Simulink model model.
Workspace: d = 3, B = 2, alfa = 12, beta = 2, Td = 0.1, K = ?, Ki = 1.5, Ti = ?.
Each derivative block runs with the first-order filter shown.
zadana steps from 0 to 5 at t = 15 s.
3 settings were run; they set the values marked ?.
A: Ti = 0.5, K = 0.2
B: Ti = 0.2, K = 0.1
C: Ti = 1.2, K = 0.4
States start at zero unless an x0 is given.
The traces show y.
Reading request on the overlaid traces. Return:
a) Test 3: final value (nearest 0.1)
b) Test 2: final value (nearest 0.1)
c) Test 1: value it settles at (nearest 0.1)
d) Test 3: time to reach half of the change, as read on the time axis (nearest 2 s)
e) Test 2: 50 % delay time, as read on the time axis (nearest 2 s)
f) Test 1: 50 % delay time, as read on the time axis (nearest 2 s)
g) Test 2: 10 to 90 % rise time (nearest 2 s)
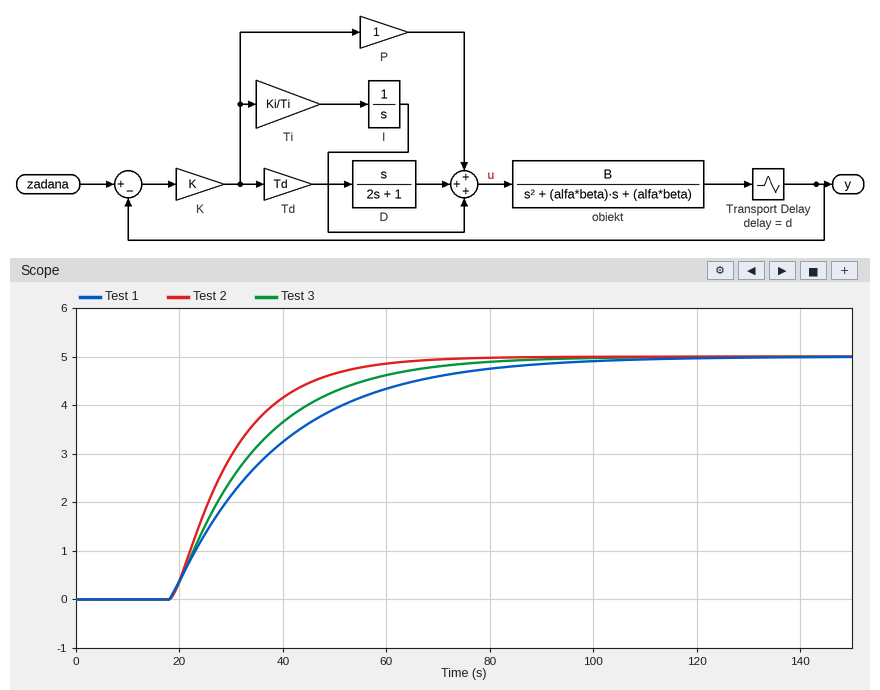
5.0
5.0
5.0
30 s
28 s
32 s
26 s
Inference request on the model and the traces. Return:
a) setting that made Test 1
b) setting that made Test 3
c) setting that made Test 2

C
A
B
